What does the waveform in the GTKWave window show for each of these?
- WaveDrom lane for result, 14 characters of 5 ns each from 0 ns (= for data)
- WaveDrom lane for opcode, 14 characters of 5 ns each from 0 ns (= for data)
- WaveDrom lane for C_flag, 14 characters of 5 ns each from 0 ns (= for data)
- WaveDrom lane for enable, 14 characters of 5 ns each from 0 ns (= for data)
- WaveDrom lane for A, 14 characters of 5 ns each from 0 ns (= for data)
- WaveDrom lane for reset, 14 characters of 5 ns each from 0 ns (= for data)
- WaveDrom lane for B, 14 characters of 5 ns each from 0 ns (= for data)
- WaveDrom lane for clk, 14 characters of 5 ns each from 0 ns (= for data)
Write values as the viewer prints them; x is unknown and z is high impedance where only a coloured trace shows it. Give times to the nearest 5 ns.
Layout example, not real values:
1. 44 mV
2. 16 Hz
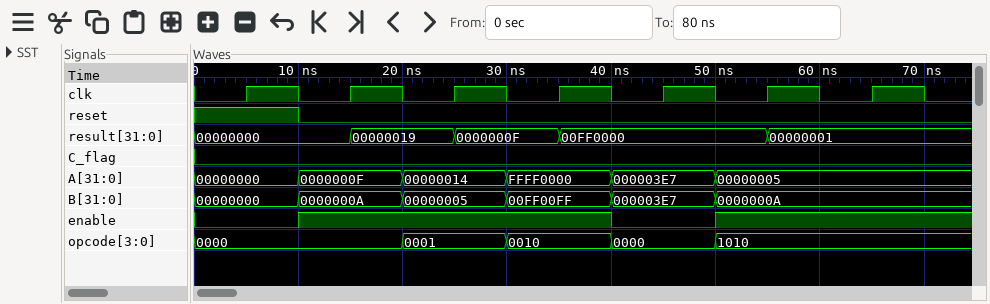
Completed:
1. {name: 'result', wave: '=..=.=.=...=..', data: '00000000 00000019 0000000F 00FF0000 00000001'}
2. {name: 'opcode', wave: '=...=.=.=.=...', data: '0000 0001 0010 0000 1010'}
3. {name: 'C_flag', wave: '0.............'}
4. {name: 'enable', wave: '0.1.....0.1...'}
5. {name: 'A', wave: '=.=.=.=.=.=...', data: '00000000 0000000F 00000014 FFFF0000 000003E7 00000005'}
6. {name: 'reset', wave: '1.0...........'}
7. {name: 'B', wave: '=.=.=.=.=.=...', data: '00000000 0000000A 00000005 00FF00FF 000003E7 0000000A'}
8. {name: 'clk', wave: '01010101010101'}
